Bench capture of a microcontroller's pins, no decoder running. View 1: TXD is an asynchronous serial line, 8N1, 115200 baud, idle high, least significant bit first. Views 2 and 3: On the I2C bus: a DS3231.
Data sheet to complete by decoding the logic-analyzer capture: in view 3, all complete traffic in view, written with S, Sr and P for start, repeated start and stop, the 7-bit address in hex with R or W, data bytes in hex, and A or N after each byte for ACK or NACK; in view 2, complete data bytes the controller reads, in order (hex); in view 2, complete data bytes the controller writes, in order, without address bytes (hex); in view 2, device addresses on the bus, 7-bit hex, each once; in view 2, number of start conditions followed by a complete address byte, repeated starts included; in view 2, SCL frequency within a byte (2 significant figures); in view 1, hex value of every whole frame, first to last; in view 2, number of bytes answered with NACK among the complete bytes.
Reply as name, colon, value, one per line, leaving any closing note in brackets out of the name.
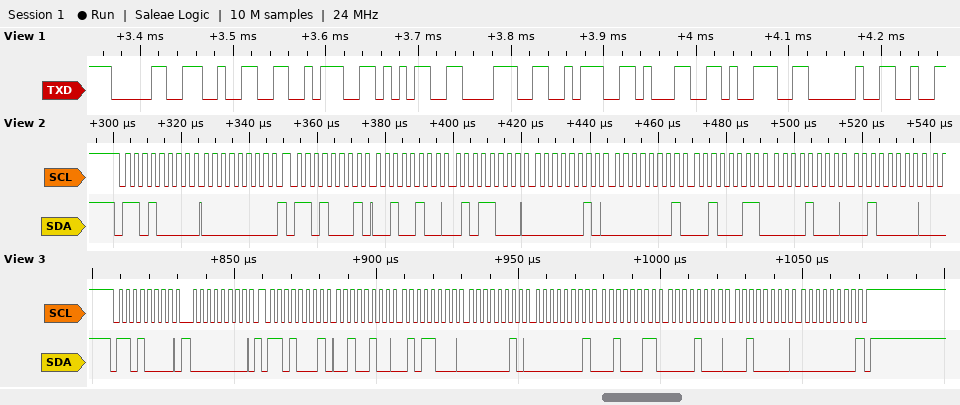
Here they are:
in view 3, all complete traffic in view, written with S, Sr and P for start, repeated start and stop, the 7-bit address in hex with R or W, data bytes in hex, and A or N after each byte for ACK or NACK: S 68W A 00 A Sr 68R A 24 A 58 A 02 A 01 A 23 A 08 A 20 A 00 N P
in view 2, complete data bytes the controller reads, in order: 24 58 02 01 23 08 20
in view 2, complete data bytes the controller writes, in order, without address bytes: 00
in view 2, device addresses on the bus, 7-bit hex, each once: 0x68
in view 2, number of start conditions followed by a complete address byte, repeated starts included: 2
in view 2, SCL frequency within a byte: 400 kHz
in view 1, hex value of every whole frame, first to last: 30 32 3A 35 38 3A 31 39 20
in view 2, number of bytes answered with NACK among the complete bytes: 0
